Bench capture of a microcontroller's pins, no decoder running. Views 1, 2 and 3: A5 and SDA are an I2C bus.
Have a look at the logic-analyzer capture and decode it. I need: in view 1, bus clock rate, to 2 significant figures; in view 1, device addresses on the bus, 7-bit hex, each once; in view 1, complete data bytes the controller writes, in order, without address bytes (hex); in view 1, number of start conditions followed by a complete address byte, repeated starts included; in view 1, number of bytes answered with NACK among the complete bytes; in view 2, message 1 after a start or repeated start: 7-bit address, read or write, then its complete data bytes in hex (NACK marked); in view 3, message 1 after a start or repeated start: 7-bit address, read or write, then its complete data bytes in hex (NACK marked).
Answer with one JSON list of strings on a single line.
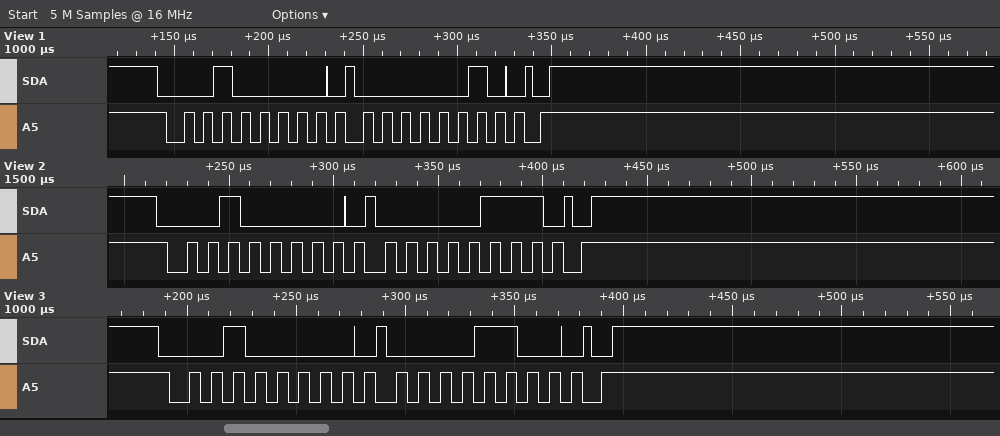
["100 kHz", "0x10", "02", "1", "0", "0x10 write: 07", "0x10 write: 0C"]
